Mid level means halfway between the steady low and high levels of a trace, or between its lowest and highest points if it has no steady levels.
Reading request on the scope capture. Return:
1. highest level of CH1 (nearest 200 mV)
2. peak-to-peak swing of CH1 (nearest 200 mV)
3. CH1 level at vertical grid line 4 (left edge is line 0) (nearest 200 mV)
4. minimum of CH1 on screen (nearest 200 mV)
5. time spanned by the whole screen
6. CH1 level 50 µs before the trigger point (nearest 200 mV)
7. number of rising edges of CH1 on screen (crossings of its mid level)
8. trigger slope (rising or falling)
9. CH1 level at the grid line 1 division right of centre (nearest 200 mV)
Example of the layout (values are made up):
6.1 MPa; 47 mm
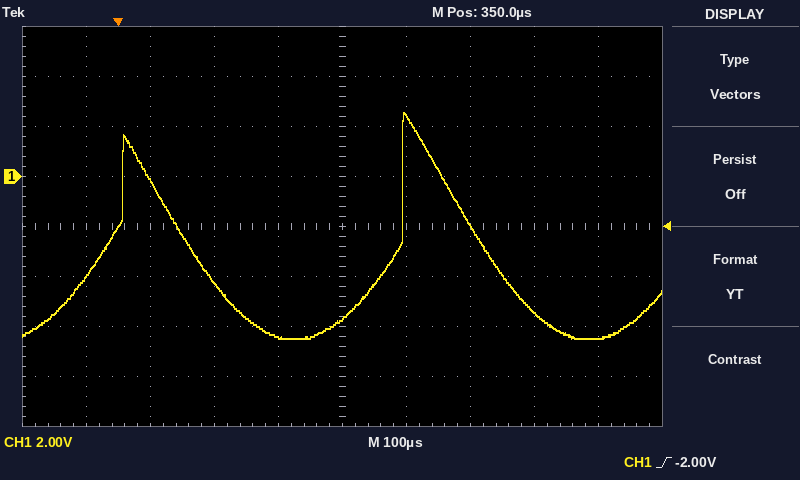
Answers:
2.6 V; 9.0 V; -6.4 V; -6.4 V; 1 ms; -4.0 V; 2; rising; 2.4 V
